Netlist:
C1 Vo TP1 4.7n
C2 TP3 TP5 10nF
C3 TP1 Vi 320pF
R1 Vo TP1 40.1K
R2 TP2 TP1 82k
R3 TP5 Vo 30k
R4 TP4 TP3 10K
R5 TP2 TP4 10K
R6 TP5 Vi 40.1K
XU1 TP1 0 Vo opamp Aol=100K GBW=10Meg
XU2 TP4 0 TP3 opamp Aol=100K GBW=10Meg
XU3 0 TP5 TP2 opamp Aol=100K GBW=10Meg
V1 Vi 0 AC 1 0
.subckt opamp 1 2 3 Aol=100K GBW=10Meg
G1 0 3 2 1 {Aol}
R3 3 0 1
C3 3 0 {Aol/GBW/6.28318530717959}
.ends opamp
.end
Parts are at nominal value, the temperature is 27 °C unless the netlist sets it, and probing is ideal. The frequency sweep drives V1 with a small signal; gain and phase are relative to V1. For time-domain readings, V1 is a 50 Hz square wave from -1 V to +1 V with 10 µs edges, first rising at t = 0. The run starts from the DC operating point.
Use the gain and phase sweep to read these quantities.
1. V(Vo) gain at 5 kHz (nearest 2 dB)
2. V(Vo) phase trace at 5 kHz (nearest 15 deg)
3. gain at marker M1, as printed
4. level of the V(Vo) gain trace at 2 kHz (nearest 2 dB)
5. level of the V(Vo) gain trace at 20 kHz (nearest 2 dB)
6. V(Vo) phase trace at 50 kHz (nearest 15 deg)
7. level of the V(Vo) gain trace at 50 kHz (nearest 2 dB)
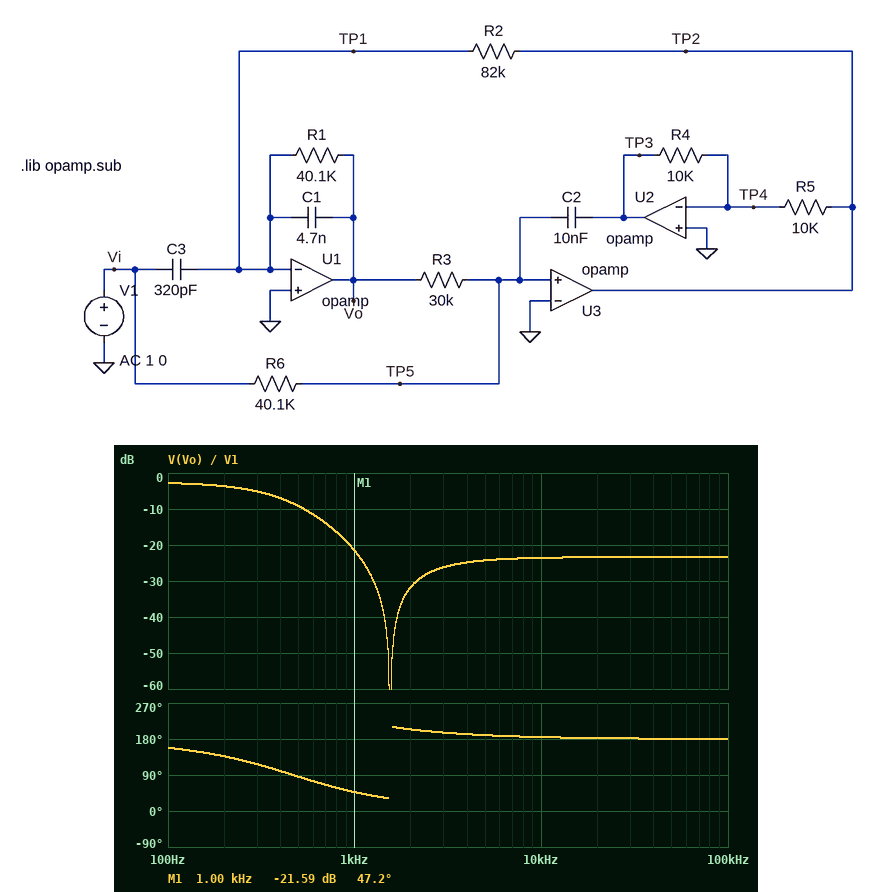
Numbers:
-24 dB
195 deg
-21.59 dB
-32 dB
-24 dB
180 deg
-24 dB
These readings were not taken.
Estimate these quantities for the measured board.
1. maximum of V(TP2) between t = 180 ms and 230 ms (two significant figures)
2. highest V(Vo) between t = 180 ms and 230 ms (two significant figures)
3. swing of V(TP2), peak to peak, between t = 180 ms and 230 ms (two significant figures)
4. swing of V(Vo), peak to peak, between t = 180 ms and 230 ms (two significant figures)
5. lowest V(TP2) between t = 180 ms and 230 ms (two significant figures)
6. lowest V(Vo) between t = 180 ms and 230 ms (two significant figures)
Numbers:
1.5 V
750 mV
3.1 V
1.5 V
-1.5 V
-750 mV
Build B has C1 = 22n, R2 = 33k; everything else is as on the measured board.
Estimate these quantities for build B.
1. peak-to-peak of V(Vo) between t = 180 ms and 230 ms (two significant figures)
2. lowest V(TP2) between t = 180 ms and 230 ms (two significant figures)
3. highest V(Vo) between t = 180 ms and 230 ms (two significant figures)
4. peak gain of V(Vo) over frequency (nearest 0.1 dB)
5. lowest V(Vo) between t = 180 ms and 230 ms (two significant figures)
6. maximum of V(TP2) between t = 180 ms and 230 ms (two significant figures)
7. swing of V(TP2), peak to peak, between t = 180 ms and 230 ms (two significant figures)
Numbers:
2.7 V
-2.0 V
1.4 V
3.2 dB
-1.4 V
2.0 V
4.0 V
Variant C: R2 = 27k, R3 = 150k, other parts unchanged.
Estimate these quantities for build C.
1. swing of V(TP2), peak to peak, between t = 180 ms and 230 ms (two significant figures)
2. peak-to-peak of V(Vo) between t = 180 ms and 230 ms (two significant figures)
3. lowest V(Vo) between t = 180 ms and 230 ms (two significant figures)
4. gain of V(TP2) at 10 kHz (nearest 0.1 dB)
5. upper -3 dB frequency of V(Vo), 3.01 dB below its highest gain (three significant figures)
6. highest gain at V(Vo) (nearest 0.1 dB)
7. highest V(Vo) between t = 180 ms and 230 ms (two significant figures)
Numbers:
5.0 V
7.5 V
-3.7 V
-28.2 dB
190 Hz
11.5 dB
3.7 V
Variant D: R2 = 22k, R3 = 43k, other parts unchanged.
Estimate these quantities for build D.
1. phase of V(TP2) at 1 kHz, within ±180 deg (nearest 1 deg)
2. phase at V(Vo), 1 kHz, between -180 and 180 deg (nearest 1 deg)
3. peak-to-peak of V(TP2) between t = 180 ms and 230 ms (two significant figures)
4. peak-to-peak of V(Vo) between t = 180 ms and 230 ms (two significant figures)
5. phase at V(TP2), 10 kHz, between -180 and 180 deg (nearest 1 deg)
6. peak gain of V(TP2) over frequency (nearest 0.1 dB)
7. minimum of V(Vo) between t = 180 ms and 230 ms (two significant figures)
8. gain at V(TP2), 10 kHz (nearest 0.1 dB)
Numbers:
-69 deg
63 deg
1.6 V
2.6 V
-90 deg
-2.7 dB
-1.3 V
-28.5 dB
